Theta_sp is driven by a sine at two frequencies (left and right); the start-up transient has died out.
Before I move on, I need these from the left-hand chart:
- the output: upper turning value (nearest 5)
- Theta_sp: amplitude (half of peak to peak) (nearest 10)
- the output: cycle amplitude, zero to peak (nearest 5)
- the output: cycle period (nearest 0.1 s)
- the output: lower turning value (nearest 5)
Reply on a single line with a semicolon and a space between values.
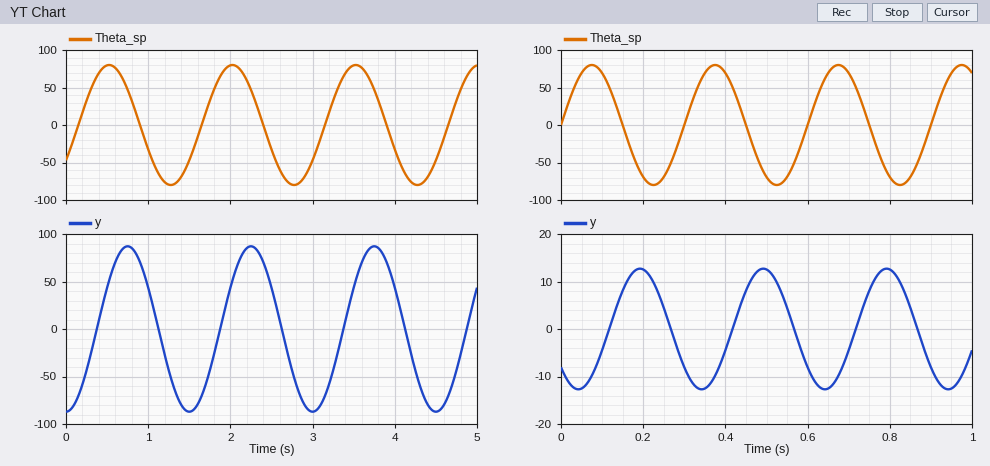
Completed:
85; 80; 85; 1.5 s; -85
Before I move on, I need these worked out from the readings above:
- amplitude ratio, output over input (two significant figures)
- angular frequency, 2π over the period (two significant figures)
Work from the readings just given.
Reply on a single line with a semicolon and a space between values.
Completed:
1.1; 4.2 rad/s
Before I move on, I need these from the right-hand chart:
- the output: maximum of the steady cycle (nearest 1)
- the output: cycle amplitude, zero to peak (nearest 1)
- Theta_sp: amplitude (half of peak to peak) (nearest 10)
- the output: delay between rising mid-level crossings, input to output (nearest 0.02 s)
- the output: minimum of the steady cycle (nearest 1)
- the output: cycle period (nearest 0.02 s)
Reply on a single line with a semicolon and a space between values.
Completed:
13; 13; 80; 0.12 s; -13; 0.30 s
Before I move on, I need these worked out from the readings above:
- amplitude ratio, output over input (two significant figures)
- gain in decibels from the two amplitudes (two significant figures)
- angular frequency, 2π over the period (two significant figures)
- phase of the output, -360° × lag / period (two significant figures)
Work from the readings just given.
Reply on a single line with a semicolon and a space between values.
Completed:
0.16; -16 dB; 21 rad/s; -140°
